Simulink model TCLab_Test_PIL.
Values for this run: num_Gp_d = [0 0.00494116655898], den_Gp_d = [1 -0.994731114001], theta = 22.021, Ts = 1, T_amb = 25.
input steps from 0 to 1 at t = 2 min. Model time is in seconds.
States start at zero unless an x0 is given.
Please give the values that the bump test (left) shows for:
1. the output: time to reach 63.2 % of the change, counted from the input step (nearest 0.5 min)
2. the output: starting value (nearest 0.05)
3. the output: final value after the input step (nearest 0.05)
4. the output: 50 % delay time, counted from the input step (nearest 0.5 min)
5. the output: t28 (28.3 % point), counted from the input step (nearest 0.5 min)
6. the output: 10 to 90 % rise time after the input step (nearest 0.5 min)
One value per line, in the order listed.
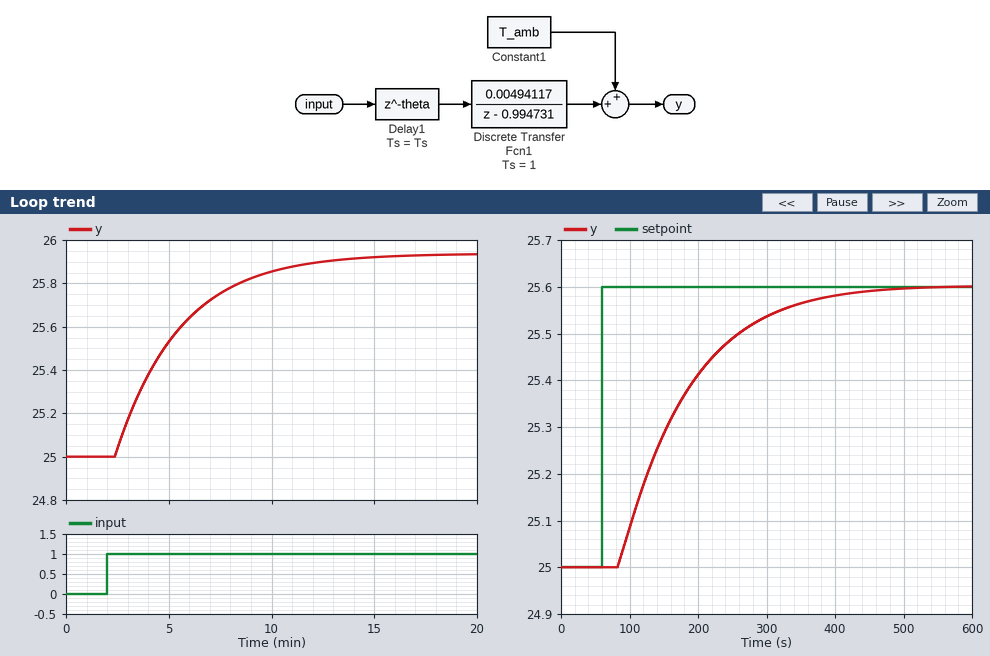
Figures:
3.5 min
25.00
25.95
2.5 min
1.5 min
7.0 min
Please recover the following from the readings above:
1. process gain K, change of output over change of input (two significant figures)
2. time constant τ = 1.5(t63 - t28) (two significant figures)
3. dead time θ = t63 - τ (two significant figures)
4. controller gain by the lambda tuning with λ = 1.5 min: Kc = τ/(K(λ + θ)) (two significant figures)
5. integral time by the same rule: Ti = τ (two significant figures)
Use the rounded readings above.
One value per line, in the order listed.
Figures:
0.95
3.0 min
0.50 min
1.6
3.0 min
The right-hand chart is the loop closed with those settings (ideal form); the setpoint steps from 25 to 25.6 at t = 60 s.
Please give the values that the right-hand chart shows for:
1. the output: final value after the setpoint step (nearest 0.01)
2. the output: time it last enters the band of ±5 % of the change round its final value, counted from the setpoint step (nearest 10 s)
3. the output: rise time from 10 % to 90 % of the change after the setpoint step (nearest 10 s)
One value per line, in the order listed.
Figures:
25.60
300 s
210 s
